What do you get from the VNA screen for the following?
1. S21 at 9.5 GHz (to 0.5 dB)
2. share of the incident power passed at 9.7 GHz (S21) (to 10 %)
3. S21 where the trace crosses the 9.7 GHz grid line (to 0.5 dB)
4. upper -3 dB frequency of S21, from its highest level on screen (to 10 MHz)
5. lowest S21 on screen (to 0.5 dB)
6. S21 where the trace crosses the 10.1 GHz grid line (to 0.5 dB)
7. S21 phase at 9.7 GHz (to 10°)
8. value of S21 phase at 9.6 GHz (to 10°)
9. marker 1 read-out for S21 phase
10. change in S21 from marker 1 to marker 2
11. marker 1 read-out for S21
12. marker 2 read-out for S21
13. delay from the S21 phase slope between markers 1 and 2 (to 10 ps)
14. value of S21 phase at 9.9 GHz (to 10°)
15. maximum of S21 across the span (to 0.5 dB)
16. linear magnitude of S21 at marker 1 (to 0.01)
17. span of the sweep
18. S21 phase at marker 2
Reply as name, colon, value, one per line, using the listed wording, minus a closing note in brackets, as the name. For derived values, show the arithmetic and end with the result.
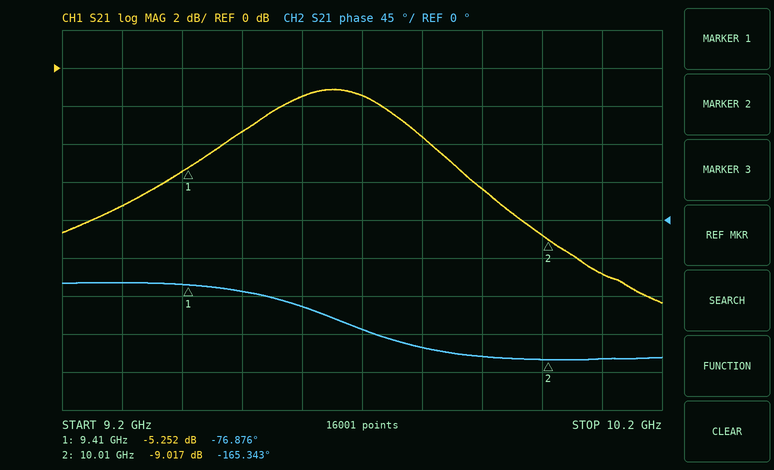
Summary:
S21 at 9.5 GHz: -3.5 dB
share of the incident power passed at 9.7 GHz (S21): 10^(-1.5/10) ≈ 70.8 %, so 70 % to the nearest 10 %
S21 where the trace crosses the 9.7 GHz grid line: -1.5 dB
upper -3 dB frequency of S21, from its highest level on screen: 9.82 GHz
lowest S21 on screen: -12.5 dB
S21 where the trace crosses the 10.1 GHz grid line: -11.0 dB
S21 phase at 9.7 GHz: -130°
value of S21 phase at 9.6 GHz: -100°
marker 1 read-out for S21 phase: -76.876°
change in S21 from marker 1 to marker 2: -9.017 − (-5.252) = -3.765 dB
marker 1 read-out for S21: -5.252 dB
marker 2 read-out for S21: -9.017 dB
delay from the S21 phase slope between markers 1 and 2: −(-165.343° − (-76.876°))/(360° × 600 MHz) ≈ 410 ps
value of S21 phase at 9.9 GHz: -160°
maximum of S21 across the span: -1.0 dB
linear magnitude of S21 at marker 1: 10^(-5.252/20) ≈ 0.55
span of the sweep: 1 GHz
S21 phase at marker 2: -165.343°
